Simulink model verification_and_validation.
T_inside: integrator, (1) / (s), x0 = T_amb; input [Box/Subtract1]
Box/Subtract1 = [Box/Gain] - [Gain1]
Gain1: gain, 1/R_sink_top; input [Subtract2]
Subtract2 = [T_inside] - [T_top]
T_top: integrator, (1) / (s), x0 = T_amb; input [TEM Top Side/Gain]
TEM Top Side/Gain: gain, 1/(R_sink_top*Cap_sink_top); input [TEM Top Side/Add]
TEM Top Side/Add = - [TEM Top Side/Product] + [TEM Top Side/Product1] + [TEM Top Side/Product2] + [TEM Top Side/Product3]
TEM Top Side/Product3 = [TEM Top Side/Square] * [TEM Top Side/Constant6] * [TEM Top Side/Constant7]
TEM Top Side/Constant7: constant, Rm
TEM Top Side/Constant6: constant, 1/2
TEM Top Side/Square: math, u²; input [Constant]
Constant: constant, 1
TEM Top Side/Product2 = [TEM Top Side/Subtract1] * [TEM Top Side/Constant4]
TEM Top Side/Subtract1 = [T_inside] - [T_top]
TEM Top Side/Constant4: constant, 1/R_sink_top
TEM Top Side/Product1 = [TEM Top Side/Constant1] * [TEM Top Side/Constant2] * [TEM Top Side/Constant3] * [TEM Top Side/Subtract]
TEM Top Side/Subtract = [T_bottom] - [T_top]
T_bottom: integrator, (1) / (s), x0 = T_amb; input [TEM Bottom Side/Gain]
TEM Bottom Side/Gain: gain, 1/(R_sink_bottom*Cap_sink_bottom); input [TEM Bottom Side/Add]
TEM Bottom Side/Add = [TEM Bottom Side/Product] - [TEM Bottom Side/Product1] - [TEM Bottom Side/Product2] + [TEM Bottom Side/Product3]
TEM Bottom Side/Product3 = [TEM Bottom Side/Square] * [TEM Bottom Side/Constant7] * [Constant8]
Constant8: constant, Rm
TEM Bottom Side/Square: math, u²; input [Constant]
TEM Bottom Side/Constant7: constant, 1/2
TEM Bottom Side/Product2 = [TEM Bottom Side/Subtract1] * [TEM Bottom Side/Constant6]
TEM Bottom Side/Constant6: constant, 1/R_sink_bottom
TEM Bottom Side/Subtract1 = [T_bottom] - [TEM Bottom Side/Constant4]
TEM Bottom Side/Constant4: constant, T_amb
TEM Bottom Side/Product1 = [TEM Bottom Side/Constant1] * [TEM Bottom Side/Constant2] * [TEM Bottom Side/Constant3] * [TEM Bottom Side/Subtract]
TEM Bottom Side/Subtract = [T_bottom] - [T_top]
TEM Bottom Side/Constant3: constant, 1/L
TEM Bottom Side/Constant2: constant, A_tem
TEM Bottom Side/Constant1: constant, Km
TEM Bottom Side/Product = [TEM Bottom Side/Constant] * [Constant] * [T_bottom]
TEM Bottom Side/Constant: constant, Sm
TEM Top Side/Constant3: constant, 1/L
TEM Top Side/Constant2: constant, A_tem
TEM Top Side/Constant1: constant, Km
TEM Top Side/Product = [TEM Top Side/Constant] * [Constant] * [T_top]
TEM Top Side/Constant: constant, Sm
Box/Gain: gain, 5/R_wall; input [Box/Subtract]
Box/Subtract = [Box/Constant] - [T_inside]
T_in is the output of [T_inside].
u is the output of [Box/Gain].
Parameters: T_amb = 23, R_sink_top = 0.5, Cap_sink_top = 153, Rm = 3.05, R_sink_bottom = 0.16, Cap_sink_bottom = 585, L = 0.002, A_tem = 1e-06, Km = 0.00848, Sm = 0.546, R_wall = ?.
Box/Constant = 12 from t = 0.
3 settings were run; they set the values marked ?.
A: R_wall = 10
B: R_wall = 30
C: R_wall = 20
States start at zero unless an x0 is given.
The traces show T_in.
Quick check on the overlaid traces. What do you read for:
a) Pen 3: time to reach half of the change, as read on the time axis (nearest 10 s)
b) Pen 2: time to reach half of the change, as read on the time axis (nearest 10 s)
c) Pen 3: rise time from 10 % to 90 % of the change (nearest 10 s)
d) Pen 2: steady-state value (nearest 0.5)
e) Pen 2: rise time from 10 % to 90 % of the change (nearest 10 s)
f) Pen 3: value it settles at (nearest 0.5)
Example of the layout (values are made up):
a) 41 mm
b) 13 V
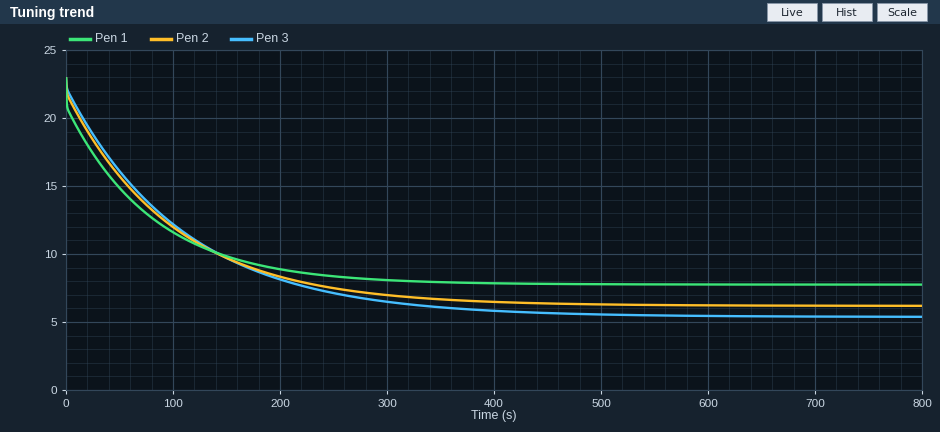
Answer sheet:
a) 70 s
b) 60 s
c) 240 s
d) 6.0
e) 220 s
f) 5.5
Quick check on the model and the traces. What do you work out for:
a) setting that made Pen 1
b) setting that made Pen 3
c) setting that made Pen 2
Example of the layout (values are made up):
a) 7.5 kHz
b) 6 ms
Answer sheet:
a) A
b) B
c) C
